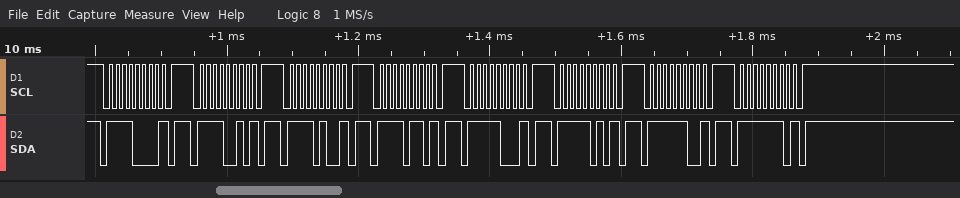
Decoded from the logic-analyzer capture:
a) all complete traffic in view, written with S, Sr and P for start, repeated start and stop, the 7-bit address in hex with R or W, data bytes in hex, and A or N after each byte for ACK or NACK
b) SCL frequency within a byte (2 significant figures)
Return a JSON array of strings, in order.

["S 78W N P S 79W N P S 7AW N P S 7BW N P S 7CW N P S 7DW N P S 7EW N P S 7FW N P", "100 kHz"]
